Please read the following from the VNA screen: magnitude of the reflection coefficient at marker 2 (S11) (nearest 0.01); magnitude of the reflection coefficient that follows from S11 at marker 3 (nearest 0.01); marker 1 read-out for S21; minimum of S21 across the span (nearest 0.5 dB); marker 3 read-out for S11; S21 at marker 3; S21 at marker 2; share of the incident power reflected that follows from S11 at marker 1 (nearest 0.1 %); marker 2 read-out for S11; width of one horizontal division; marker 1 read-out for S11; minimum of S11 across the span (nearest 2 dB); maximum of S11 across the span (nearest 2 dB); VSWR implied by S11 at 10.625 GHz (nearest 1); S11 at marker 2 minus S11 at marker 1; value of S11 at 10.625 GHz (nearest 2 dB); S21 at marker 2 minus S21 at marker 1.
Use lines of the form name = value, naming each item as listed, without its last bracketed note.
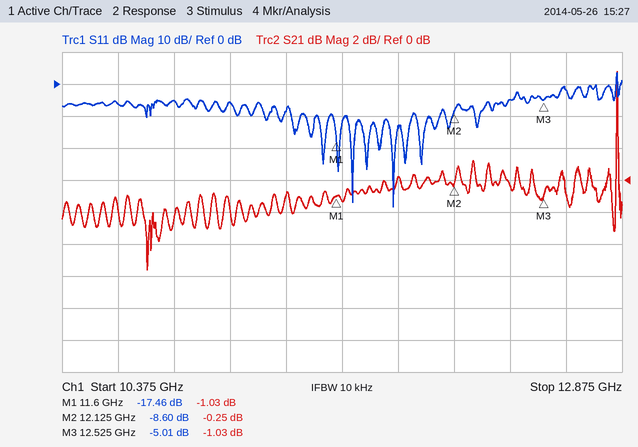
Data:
magnitude of the reflection coefficient at marker 2 (S11) = 0.37
magnitude of the reflection coefficient that follows from S11 at marker 3 = 0.56
marker 1 read-out for S21 = -1.03 dB
minimum of S21 across the span = -5.5 dB
marker 3 read-out for S11 = -5.01 dB
S21 at marker 3 = -1.03 dB
S21 at marker 2 = -0.25 dB
share of the incident power reflected that follows from S11 at marker 1 = 1.8 %
marker 2 read-out for S11 = -8.60 dB
width of one horizontal division = 250 MHz
marker 1 read-out for S11 = -17.46 dB
minimum of S11 across the span = -38 dB
maximum of S11 across the span = 4 dB
VSWR implied by S11 at 10.625 GHz = 3
S11 at marker 2 minus S11 at marker 1 = 8.86 dB
value of S11 at 10.625 GHz = -6 dB
S21 at marker 2 minus S21 at marker 1 = 0.78 dB
